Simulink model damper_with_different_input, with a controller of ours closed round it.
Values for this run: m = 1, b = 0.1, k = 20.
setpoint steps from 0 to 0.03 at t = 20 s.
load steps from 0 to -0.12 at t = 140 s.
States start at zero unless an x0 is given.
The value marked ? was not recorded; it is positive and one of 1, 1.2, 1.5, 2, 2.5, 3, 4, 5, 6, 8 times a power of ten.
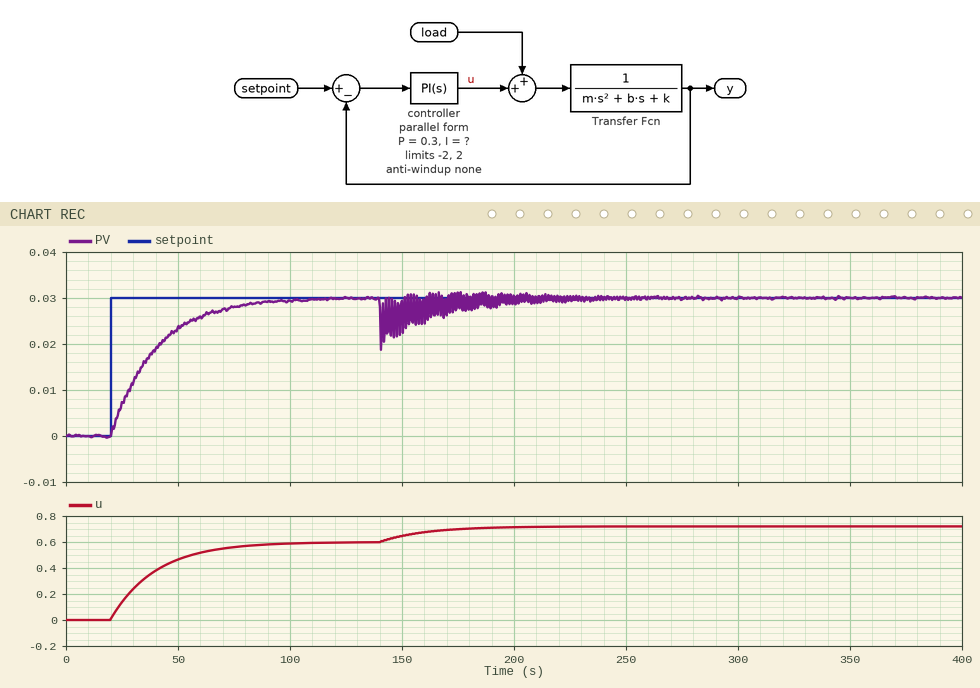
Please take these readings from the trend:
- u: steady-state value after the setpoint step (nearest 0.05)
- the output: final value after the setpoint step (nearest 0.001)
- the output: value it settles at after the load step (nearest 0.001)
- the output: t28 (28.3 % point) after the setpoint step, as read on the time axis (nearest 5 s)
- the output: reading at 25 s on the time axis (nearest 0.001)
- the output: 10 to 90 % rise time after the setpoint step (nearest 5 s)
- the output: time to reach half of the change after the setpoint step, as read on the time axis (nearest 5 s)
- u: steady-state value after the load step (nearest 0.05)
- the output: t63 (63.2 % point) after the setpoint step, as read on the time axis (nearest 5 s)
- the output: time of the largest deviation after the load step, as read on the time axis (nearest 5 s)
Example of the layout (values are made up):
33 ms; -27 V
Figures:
0.60; 0.030; 0.030; 25 s; 0.007; 45 s; 35 s; 0.70; 40 s; 140 s
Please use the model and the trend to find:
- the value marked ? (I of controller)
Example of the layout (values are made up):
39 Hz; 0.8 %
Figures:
1
